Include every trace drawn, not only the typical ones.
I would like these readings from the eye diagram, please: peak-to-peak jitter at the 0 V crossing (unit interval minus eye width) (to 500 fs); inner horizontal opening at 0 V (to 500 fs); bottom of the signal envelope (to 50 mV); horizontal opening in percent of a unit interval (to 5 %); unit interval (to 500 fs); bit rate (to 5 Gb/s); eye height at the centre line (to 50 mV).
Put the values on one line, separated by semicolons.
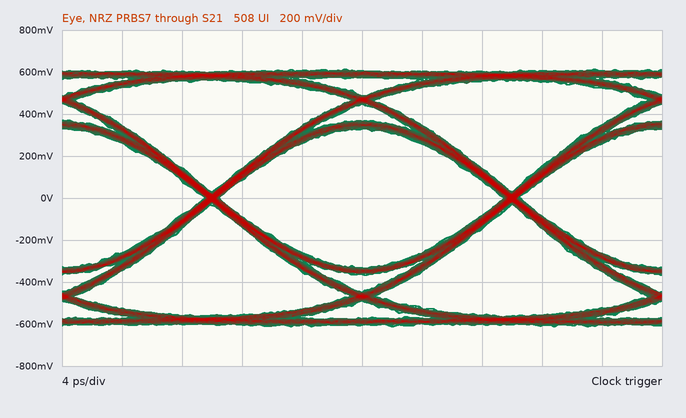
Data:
1.0 ps; 19.0 ps; -600 mV; 95 %; 20.0 ps; 50 Gb/s; 650 mV
